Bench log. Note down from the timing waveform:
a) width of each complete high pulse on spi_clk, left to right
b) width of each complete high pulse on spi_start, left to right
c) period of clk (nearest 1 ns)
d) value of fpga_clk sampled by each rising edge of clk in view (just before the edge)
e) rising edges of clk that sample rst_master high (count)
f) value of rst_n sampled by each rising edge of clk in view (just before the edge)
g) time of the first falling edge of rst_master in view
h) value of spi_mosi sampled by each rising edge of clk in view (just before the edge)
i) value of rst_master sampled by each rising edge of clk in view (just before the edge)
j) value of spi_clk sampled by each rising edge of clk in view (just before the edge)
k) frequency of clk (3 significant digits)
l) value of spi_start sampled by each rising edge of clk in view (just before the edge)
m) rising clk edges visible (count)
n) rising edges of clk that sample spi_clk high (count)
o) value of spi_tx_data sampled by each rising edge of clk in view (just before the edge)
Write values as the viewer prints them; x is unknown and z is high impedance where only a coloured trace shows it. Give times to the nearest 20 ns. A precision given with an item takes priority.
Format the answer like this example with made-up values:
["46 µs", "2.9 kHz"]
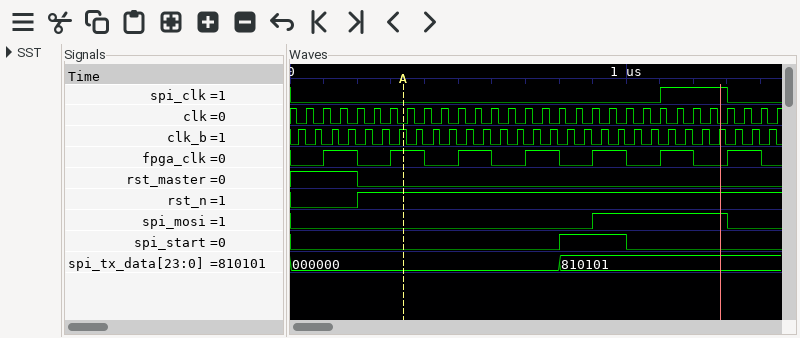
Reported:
["200 ns", "200 ns", "50 ns", "0 0 1 1 0 0 1 1 0 0 1 1 0 0 1 1 0 0 1 1 0 0 1 1 0 0 1 1 0", "4", "0 0 0 0 1 1 1 1 1 1 1 1 1 1 1 1 1 1 1 1 1 1 1 1 1 1 1 1 1", "200 ns", "0 0 0 0 0 0 0 0 0 0 0 0 0 0 0 0 0 0 1 1 1 1 1 1 1 1 0 0 0", "1 1 1 1 0 0 0 0 0 0 0 0 0 0 0 0 0 0 0 0 0 0 0 0 0 0 0 0 0", "0 0 0 0 0 0 0 0 0 0 0 0 0 0 0 0 0 0 0 0 0 0 1 1 1 1 0 0 0", "20.0 MHz", "0 0 0 0 0 0 0 0 0 0 0 0 0 0 0 0 1 1 1 1 0 0 0 0 0 0 0 0 0", "29", "4", "000000, 000000, 000000, 000000, 000000, 000000, 000000, 000000, 000000, 000000, 000000, 000000, 000000, 000000, 000000, 000000, 810101, 810101, 810101, 810101, 810101, 810101, 810101, 810101, 810101, 810101, 810101, 810101, 810101"]
